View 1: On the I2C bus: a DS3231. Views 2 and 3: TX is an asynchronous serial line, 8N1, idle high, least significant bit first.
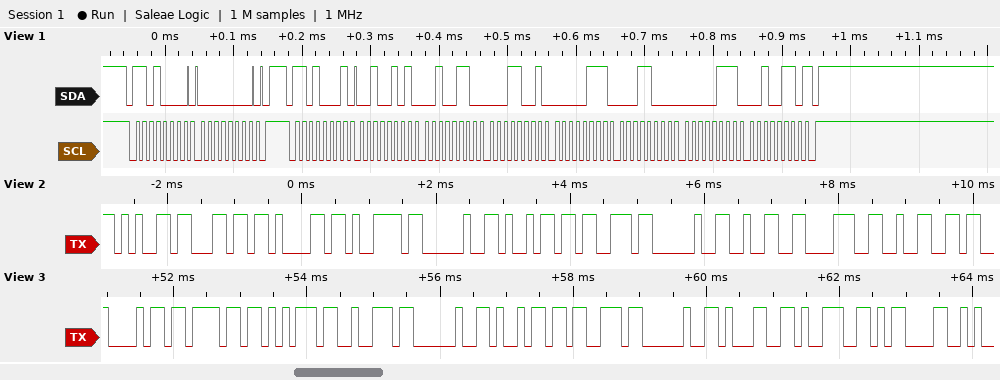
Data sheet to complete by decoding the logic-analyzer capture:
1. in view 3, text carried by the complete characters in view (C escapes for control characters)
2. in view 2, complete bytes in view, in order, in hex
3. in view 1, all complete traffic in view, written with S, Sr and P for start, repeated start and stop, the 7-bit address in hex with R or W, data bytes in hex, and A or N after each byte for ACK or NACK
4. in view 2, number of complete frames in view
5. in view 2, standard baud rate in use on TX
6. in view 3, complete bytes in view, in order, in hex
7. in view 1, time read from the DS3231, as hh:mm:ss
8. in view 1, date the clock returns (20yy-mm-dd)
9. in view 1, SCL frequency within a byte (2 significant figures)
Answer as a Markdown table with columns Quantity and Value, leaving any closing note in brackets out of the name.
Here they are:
| Quantity | Value |
|---|---|
| in view 3, text carried by the complete characters in view | "hour is 19\r" |
| in view 2, complete bytes in view, in order, in hex | 65 6C 61 79 20 69 73 20 32 38 32 |
| in view 1, all complete traffic in view, written with S, Sr and P for start, repeated start and stop, the 7-bit address in hex with R or W, data bytes in hex, and A or N after each byte for ACK or NACK | S 68W A 00 A P S 68R A 25 A 26 A 19 A 07 A 18 A 07 A 26 N P |
| in view 2, number of complete frames in view | 11 |
| in view 2, standard baud rate in use on TX | 9600 baud |
| in view 3, complete bytes in view, in order, in hex | 68 6F 75 72 20 69 73 20 31 39 0D |
| in view 1, time read from the DS3231, as hh:mm:ss | 19:26:25 |
| in view 1, date the clock returns | 2026-07-18 |
| in view 1, SCL frequency within a byte | 100 kHz |
